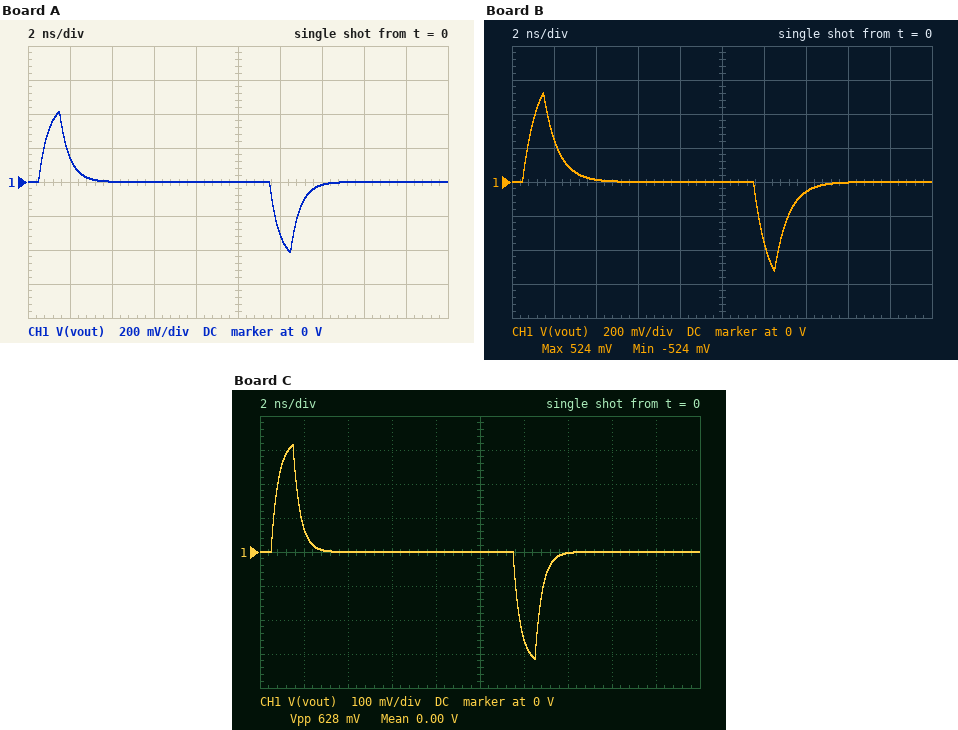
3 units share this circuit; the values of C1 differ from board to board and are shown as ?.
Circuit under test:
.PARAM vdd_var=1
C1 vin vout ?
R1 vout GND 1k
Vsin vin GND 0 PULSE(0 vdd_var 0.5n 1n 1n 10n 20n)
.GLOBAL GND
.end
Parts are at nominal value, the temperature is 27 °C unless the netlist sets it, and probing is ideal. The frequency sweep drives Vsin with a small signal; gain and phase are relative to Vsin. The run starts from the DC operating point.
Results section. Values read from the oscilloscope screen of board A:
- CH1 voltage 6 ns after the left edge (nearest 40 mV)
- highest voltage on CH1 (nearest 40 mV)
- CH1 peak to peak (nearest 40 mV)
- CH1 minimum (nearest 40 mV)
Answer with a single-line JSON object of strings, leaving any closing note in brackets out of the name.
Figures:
{"CH1 voltage 6 ns after the left edge": "0 V", "highest voltage on CH1": "400 mV", "CH1 peak to peak": "840 mV", "CH1 minimum": "-400 mV"}
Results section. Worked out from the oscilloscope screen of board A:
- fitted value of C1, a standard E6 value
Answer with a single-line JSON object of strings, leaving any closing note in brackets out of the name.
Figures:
{"fitted value of C1, a standard E6 value": "470 fF"}
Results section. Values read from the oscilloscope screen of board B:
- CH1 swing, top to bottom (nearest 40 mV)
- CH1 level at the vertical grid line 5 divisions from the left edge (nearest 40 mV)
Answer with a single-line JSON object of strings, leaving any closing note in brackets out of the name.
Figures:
{"CH1 swing, top to bottom": "1.04 V", "CH1 level at the vertical grid line 5 divisions from the left edge": "0 V"}
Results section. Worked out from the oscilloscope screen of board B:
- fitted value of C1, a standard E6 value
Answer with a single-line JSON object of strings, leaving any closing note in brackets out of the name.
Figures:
{"fitted value of C1, a standard E6 value": "680 fF"}
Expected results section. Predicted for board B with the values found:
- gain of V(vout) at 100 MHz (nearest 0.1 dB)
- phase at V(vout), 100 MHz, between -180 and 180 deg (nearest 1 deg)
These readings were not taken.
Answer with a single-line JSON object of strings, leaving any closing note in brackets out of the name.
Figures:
{"gain of V(vout) at 100 MHz": "-8.1 dB", "phase at V(vout), 100 MHz, between -180 and 180 deg": "67 deg"}
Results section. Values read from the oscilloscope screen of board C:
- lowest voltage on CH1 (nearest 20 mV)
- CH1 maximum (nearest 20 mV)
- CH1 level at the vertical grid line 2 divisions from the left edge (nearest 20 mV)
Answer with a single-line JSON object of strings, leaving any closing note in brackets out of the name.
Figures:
{"lowest voltage on CH1": "-320 mV", "CH1 maximum": "320 mV", "CH1 level at the vertical grid line 2 divisions from the left edge": "0 V"}
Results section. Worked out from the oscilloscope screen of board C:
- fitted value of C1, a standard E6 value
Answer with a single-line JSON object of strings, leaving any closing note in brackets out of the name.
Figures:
{"fitted value of C1, a standard E6 value": "330 fF"}
